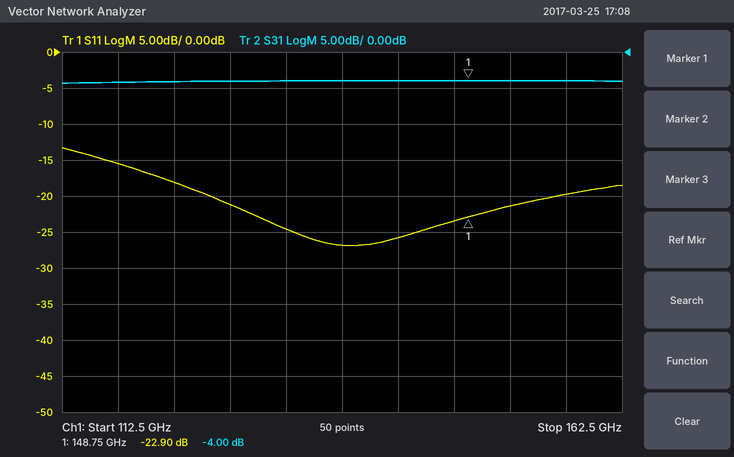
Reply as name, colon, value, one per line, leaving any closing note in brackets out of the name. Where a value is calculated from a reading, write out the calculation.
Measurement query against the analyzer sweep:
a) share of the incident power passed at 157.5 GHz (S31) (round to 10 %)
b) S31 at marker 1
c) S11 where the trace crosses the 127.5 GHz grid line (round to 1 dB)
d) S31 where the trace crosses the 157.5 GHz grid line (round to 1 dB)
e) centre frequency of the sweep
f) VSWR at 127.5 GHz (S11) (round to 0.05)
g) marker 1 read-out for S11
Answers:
share of the incident power passed at 157.5 GHz (S31): 10^(-4/10) ≈ 40 %
S31 at marker 1: -4.00 dB
S11 where the trace crosses the 127.5 GHz grid line: -21 dB
S31 where the trace crosses the 157.5 GHz grid line: -4 dB
centre frequency of the sweep: 137.5 GHz
VSWR at 127.5 GHz (S11): |Γ| = 10^(-21/20) = 0.0891; VSWR = (1 + 0.0891)/(1 − 0.0891) ≈ 1.20
marker 1 read-out for S11: -22.90 dB
